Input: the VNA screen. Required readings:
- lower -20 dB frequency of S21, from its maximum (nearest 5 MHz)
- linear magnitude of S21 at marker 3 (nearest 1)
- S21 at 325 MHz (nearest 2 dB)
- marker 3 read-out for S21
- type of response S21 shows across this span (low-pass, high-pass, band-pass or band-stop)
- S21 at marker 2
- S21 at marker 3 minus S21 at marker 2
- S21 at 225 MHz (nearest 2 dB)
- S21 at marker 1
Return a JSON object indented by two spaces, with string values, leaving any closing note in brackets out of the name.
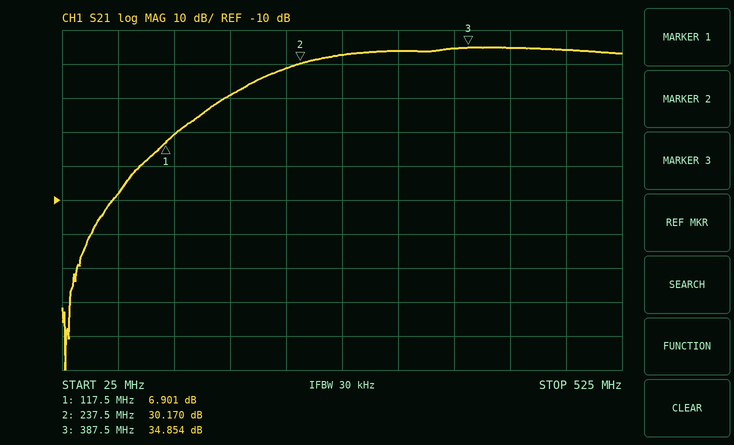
{
  "lower -20 dB frequency of S21, from its maximum": "150 MHz",
  "linear magnitude of S21 at marker 3": "55",
  "S21 at 325 MHz": "34 dB",
  "marker 3 read-out for S21": "34.854 dB",
  "type of response S21 shows across this span": "high-pass",
  "S21 at marker 2": "30.170 dB",
  "S21 at marker 3 minus S21 at marker 2": "4.684 dB",
  "S21 at 225 MHz": "28 dB",
  "S21 at marker 1": "6.901 dB"
}
